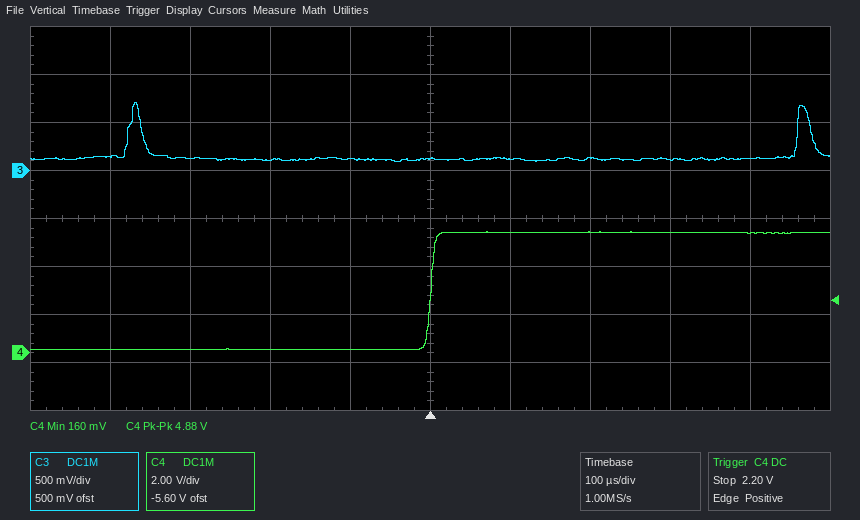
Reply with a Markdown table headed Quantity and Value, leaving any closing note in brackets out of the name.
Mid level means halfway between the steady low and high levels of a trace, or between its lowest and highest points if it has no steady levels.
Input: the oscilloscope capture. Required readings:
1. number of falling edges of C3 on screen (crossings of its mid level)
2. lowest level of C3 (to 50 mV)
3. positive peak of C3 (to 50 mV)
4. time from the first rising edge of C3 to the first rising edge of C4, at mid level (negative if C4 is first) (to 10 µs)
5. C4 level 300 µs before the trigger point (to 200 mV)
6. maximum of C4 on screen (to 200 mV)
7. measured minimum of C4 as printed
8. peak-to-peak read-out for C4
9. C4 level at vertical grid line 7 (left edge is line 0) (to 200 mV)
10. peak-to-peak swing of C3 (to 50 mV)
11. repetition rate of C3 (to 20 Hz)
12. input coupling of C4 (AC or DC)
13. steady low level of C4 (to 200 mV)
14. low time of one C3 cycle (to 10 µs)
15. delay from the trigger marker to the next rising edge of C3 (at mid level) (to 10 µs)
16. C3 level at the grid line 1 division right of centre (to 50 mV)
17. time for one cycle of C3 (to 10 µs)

| Quantity | Value |
|---|---|
| number of falling edges of C3 on screen | 2 |
| lowest level of C3 | 100 mV |
| positive peak of C3 | 700 mV |
| time from the first rising edge of C3 to the first rising edge of C4, at mid level (negative if C4 is first) | +380 µs |
| C4 level 300 µs before the trigger point | 200 mV |
| maximum of C4 on screen | 5.0 V |
| measured minimum of C4 as printed | 160 mV |
| peak-to-peak read-out for C4 | 4.88 V |
| C4 level at vertical grid line 7 (left edge is line 0) | 5.0 V |
| peak-to-peak swing of C3 | 600 mV |
| repetition rate of C3 | 1.20 kHz |
| input coupling of C4 | DC |
| steady low level of C4 | 200 mV |
| low time of one C3 cycle | 820 µs |
| delay from the trigger marker to the next rising edge of C3 (at mid level) | 460 µs |
| C3 level at the grid line 1 division right of centre | 100 mV |
| time for one cycle of C3 | 840 µs |
